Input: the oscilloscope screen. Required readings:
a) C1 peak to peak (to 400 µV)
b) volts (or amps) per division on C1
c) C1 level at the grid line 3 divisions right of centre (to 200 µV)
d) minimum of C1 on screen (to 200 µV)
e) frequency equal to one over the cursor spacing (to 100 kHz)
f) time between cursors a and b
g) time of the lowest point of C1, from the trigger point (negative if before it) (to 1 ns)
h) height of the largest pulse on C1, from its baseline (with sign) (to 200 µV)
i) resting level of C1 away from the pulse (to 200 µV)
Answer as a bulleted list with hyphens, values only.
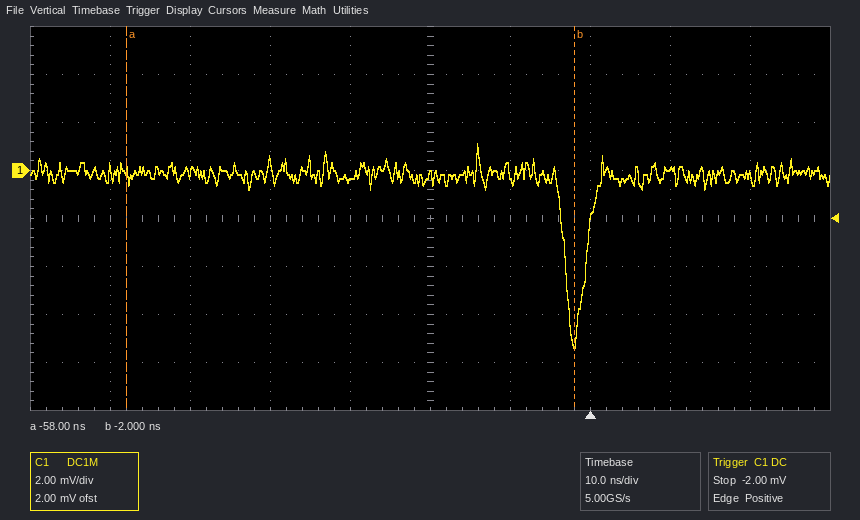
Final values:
- 8.4 mV
- 2 mV
- 0.0 mV
- -7.4 mV
- 17.9 MHz
- 56 ns
- -2 ns
- -7.2 mV
- -200 µV
